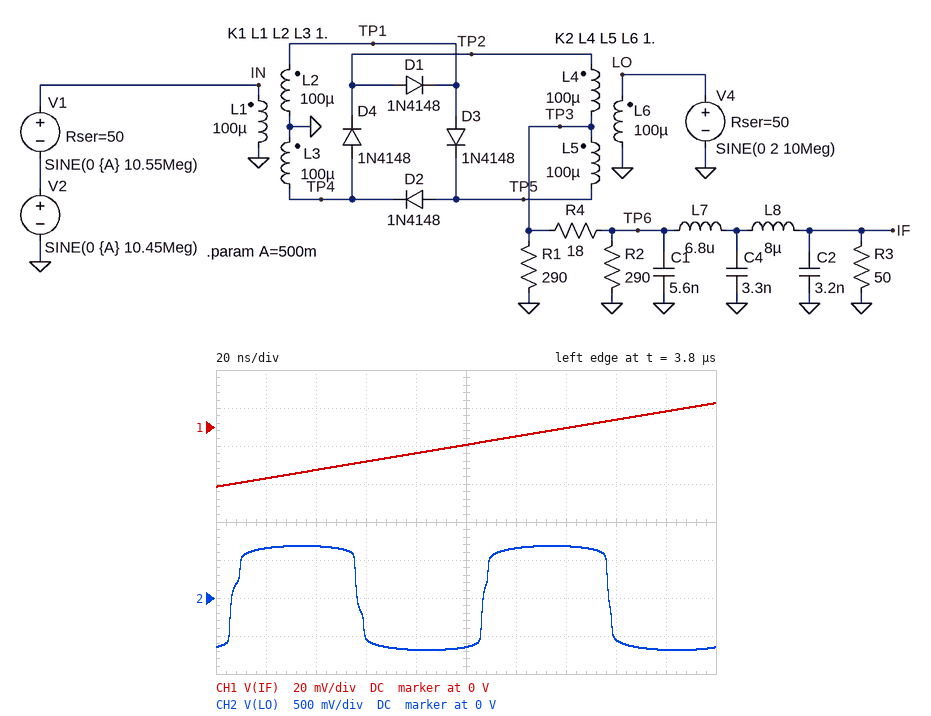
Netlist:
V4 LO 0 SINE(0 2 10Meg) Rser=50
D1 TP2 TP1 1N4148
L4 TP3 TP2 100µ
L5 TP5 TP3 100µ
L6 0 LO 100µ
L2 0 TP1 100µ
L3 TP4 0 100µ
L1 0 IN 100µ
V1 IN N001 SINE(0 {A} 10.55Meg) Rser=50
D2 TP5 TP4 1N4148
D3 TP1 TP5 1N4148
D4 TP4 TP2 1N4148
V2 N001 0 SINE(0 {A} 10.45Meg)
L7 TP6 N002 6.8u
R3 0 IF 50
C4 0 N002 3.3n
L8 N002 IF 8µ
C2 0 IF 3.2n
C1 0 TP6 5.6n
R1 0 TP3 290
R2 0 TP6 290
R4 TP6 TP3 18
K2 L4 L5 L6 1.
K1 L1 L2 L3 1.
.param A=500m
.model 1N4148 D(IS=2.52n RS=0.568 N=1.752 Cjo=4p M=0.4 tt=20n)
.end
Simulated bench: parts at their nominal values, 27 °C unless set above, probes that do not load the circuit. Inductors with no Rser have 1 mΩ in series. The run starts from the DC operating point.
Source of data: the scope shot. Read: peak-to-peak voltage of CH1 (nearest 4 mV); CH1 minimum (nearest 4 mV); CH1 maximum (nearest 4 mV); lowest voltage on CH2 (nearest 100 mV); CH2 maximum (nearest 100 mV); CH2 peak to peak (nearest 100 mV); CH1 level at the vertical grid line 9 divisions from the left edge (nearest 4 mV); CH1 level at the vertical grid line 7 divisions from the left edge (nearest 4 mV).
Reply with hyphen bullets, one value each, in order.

- 44 mV
- -32 mV
- 12 mV
- -700 mV
- 700 mV
- 1.4 V
- 8 mV
- 0 V
